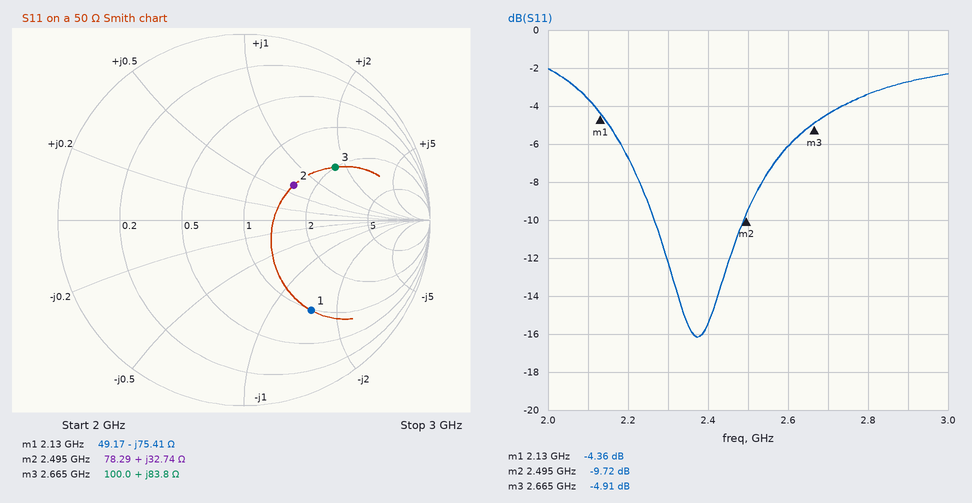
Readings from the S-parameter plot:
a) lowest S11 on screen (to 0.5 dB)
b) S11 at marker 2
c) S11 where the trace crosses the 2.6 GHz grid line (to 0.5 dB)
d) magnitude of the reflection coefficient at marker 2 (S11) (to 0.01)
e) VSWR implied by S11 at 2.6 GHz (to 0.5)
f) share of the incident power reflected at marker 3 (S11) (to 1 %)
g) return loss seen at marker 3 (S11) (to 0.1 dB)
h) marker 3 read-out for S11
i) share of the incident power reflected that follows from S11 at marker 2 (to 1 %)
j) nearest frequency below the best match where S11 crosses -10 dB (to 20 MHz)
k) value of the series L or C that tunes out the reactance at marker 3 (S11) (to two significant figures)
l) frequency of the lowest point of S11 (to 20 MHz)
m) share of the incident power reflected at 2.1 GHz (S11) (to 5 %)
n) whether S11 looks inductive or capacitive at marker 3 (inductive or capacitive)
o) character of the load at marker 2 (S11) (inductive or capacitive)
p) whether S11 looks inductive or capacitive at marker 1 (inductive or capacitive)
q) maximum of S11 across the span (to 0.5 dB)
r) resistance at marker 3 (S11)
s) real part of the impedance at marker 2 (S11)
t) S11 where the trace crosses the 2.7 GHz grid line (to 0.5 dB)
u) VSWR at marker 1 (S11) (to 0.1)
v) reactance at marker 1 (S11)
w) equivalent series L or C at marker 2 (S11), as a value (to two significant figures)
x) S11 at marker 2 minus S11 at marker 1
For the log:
-16.0 dB
-9.72 dB
-6.0 dB
0.33
3.0
32 %
4.9 dB
-4.91 dB
11 %
2.26 GHz
710 fF
2.38 GHz
45 %
inductive
inductive
capacitive
-2.0 dB
100.0 Ω
78.29 Ω
-4.5 dB
4.1
-75.41 Ω
2.1 nH
-5.36 dB
